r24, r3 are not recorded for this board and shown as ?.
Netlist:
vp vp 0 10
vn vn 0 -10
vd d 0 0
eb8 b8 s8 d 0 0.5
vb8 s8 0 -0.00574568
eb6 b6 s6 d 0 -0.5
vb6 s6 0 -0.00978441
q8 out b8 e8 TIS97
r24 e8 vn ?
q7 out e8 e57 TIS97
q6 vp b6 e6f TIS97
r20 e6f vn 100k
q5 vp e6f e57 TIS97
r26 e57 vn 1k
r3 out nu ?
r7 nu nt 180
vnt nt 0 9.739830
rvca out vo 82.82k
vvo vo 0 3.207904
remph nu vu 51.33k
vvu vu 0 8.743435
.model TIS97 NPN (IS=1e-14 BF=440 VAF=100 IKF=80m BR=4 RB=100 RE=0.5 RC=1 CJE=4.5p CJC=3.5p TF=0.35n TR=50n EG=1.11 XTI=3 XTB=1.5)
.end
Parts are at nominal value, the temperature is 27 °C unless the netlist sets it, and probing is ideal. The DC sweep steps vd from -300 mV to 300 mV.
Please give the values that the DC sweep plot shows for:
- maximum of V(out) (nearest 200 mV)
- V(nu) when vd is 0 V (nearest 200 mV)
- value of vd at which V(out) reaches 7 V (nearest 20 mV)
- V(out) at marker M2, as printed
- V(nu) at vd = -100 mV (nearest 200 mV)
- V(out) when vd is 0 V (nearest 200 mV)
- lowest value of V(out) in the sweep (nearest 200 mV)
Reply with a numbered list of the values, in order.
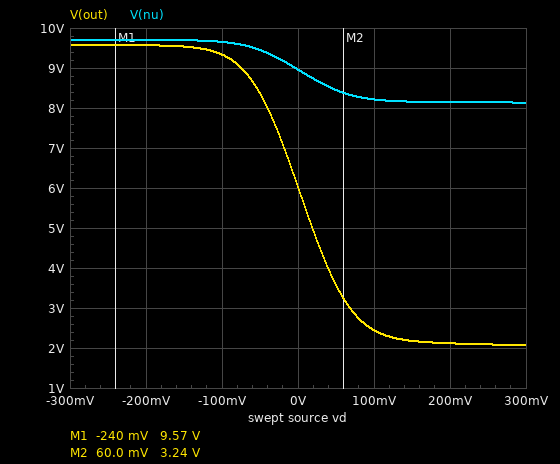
1. 9.6 V
2. 9.0 V
3. -20 mV
4. 3.24 V
5. 9.6 V
6. 6.0 V
7. 2.0 V
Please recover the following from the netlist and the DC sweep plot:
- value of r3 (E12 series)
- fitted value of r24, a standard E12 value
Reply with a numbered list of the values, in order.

1. 680 Ω
2. 82 kΩ
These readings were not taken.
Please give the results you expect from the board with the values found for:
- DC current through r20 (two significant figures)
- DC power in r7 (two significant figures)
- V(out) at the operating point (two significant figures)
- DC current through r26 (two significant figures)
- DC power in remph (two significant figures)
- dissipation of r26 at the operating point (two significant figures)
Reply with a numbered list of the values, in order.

1. 94 µA
2. 3.4 mW
3. 6.0 V
4. 8.7 mA
5. 930 nW
6. 76 mW
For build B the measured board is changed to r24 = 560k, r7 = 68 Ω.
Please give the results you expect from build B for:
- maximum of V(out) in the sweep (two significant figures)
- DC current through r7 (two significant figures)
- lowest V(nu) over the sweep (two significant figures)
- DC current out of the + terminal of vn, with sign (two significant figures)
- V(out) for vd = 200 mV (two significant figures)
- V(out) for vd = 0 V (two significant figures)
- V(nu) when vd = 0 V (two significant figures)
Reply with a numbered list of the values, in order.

1. 9.7 V
2. 6.5 mA
3. 9.1 V
4. -8.8 mA
5. 3.1 V
6. 4.9 V
7. 9.3 V
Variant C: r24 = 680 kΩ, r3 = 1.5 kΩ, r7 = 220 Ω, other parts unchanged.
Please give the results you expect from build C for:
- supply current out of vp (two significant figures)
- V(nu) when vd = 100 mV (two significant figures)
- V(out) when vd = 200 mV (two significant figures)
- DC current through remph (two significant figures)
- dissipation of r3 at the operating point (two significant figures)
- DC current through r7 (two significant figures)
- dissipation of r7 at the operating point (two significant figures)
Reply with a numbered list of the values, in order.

1. 2.8 mA
2. 8.4 V
3. -660 mV
4. 6.2 µA
5. 54 mW
6. 6.0 mA
7. 7.8 mW
